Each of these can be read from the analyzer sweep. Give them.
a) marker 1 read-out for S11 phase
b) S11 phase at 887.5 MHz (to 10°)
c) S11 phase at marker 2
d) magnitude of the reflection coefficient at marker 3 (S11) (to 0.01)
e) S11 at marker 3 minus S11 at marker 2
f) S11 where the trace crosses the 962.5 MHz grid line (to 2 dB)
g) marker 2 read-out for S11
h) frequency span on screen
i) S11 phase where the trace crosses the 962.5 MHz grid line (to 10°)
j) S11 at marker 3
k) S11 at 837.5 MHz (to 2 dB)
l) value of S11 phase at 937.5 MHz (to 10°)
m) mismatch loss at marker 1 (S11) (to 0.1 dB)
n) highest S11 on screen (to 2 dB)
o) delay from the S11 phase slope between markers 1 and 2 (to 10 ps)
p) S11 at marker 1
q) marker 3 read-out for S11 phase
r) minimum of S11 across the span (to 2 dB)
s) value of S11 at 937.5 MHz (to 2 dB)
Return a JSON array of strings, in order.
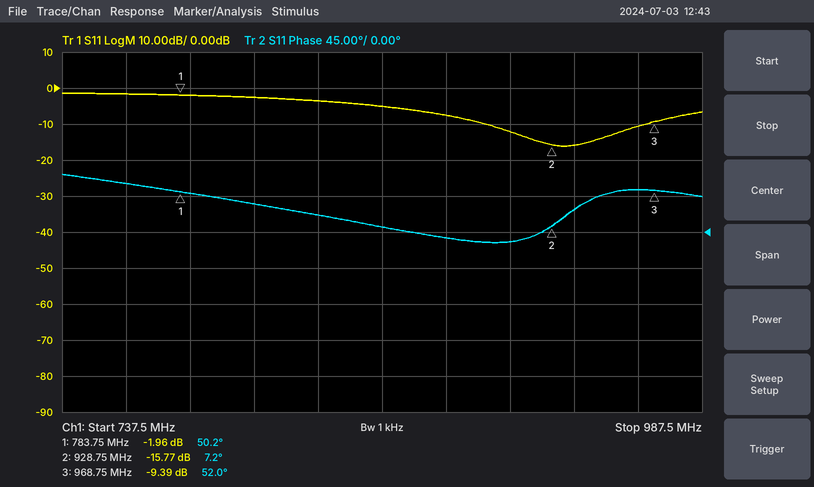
["50.2°", "-10°", "7.2°", "0.34", "6.38 dB", "-10 dB", "-15.77 dB", "250 MHz", "50°", "-9.39 dB", "-4 dB", "30°", "4.4 dB", "-2 dB", "820 ps", "-1.96 dB", "52.0°", "-16 dB", "-16 dB"]
